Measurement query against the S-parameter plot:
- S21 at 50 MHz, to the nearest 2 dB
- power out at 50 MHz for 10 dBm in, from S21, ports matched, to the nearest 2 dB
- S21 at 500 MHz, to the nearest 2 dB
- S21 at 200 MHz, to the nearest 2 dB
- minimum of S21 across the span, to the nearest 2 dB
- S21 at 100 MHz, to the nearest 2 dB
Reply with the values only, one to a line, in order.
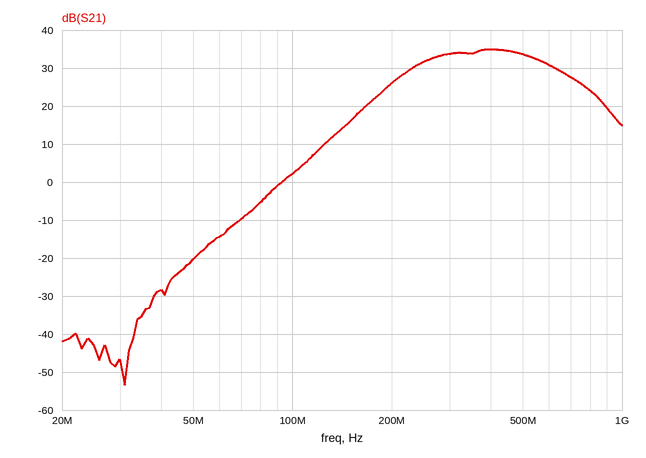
-20 dB
-10 dBm
34 dB
26 dB
-54 dB
2 dB
